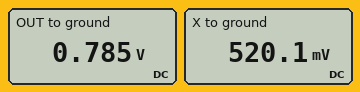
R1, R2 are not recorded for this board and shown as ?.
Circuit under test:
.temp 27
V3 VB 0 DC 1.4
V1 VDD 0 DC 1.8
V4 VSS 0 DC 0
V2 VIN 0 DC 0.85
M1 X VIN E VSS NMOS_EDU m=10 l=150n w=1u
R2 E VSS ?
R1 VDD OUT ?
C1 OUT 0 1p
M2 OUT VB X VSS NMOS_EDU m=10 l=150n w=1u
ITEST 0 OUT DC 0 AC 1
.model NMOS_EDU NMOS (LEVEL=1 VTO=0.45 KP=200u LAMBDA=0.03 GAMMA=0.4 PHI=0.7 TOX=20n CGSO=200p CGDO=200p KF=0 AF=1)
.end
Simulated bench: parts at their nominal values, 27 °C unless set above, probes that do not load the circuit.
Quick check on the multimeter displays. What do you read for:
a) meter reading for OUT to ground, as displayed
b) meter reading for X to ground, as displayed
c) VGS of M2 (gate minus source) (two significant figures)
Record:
0.785 V
520.1 mV
880 mV
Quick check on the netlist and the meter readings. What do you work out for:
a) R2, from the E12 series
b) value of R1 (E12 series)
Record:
100 Ω
1.5 kΩ
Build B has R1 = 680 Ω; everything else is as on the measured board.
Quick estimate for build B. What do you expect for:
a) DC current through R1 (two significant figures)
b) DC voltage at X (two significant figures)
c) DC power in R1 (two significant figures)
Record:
680 µA
530 mV
310 µW
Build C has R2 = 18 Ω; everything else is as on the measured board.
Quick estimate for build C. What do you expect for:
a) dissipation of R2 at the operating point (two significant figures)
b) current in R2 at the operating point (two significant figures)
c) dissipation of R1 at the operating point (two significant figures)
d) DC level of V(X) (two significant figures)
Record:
15 µW
910 µA
1.2 mW
300 mV
